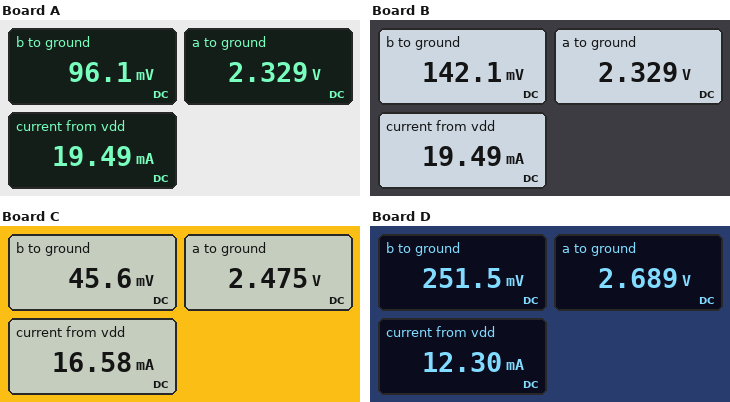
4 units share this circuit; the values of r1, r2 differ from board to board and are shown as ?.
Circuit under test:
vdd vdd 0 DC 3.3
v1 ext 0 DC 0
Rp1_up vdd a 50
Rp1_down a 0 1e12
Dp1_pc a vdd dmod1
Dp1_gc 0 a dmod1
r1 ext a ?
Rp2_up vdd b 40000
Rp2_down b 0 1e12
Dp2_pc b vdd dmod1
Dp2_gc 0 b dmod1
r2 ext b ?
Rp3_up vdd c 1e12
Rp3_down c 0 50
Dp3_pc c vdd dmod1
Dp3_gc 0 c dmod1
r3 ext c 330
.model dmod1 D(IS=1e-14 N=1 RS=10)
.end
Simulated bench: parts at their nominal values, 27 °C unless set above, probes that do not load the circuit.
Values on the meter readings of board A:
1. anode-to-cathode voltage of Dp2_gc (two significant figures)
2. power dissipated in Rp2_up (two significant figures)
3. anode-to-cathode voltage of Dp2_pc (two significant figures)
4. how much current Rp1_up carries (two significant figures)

-96 mV
260 µW
-3.2 V
19 mA
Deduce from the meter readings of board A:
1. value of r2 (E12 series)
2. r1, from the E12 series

1.2 kΩ
120 Ω
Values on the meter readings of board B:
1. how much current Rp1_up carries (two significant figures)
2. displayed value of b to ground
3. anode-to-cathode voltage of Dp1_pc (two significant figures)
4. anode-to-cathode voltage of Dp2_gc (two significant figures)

19 mA
142.1 mV
-970 mV
-140 mV
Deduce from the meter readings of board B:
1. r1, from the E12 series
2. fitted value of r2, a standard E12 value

120 Ω
1.8 kΩ
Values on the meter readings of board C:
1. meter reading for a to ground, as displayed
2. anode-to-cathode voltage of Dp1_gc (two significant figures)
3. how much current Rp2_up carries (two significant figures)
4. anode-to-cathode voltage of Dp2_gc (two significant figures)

2.475 V
-2.5 V
81 µA
-46 mV
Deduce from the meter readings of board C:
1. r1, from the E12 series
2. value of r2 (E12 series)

150 Ω
560 Ω
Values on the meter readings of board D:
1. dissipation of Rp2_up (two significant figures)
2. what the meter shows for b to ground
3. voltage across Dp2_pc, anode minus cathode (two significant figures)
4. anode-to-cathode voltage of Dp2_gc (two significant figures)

230 µW
251.5 mV
-3.0 V
-250 mV
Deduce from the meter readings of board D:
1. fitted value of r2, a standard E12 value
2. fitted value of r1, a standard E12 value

3.3 kΩ
220 Ω
